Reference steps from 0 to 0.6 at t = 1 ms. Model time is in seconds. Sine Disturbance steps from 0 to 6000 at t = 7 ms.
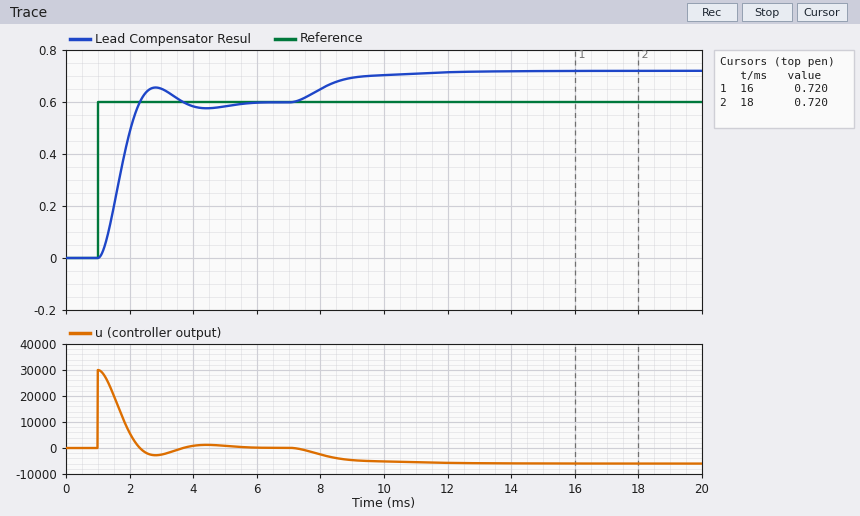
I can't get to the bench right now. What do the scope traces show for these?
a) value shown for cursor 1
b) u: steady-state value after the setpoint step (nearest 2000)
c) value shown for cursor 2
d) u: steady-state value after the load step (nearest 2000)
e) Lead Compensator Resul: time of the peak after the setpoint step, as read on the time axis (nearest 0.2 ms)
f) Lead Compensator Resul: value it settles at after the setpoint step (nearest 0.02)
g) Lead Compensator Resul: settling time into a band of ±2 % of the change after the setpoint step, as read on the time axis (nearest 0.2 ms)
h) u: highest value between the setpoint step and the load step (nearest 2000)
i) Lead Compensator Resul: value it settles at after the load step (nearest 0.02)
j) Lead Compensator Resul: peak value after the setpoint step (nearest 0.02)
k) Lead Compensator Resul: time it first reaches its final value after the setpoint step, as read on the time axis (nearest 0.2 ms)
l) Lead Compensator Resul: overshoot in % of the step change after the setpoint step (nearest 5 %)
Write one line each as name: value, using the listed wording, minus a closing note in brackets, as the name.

value shown for cursor 1: 0.720
u: steady-state value after the setpoint step: 0
value shown for cursor 2: 0.720
u: steady-state value after the load step: -6000
Lead Compensator Resul: time of the peak after the setpoint step, as read on the time axis: 2.8 ms
Lead Compensator Resul: value it settles at after the setpoint step: 0.60
Lead Compensator Resul: settling time into a band of ±2 % of the change after the setpoint step, as read on the time axis: 5.2 ms
u: highest value between the setpoint step and the load step: 30000
Lead Compensator Resul: value it settles at after the load step: 0.72
Lead Compensator Resul: peak value after the setpoint step: 0.66
Lead Compensator Resul: time it first reaches its final value after the setpoint step, as read on the time axis: 2.4 ms
Lead Compensator Resul: overshoot in % of the step change after the setpoint step: 10 %
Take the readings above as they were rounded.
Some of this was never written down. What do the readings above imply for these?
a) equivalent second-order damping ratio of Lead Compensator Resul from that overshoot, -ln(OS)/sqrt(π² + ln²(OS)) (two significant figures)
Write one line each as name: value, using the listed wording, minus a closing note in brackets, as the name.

equivalent second-order damping ratio of Lead Compensator Resul from that overshoot, -ln(OS)/sqrt(π² + ln²(OS)): 0.59
